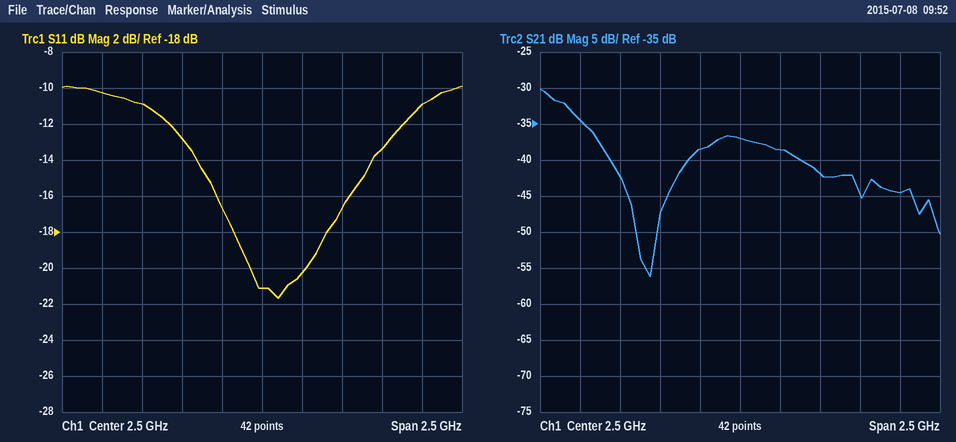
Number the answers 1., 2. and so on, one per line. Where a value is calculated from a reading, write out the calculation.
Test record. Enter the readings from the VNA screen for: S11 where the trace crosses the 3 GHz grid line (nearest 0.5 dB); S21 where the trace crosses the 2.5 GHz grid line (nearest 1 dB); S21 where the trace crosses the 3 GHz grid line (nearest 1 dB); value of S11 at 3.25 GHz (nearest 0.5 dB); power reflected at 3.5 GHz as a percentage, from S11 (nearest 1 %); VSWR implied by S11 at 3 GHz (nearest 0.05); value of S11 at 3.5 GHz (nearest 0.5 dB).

1. -16.5 dB
2. -37 dB
3. -42 dB
4. -13.5 dB
5. 10^(-11/10) ≈ 8 %
6. |Γ| = 10^(-16.5/20) = 0.1496; VSWR = (1 + 0.1496)/(1 − 0.1496) ≈ 1.35
7. -11.0 dB
